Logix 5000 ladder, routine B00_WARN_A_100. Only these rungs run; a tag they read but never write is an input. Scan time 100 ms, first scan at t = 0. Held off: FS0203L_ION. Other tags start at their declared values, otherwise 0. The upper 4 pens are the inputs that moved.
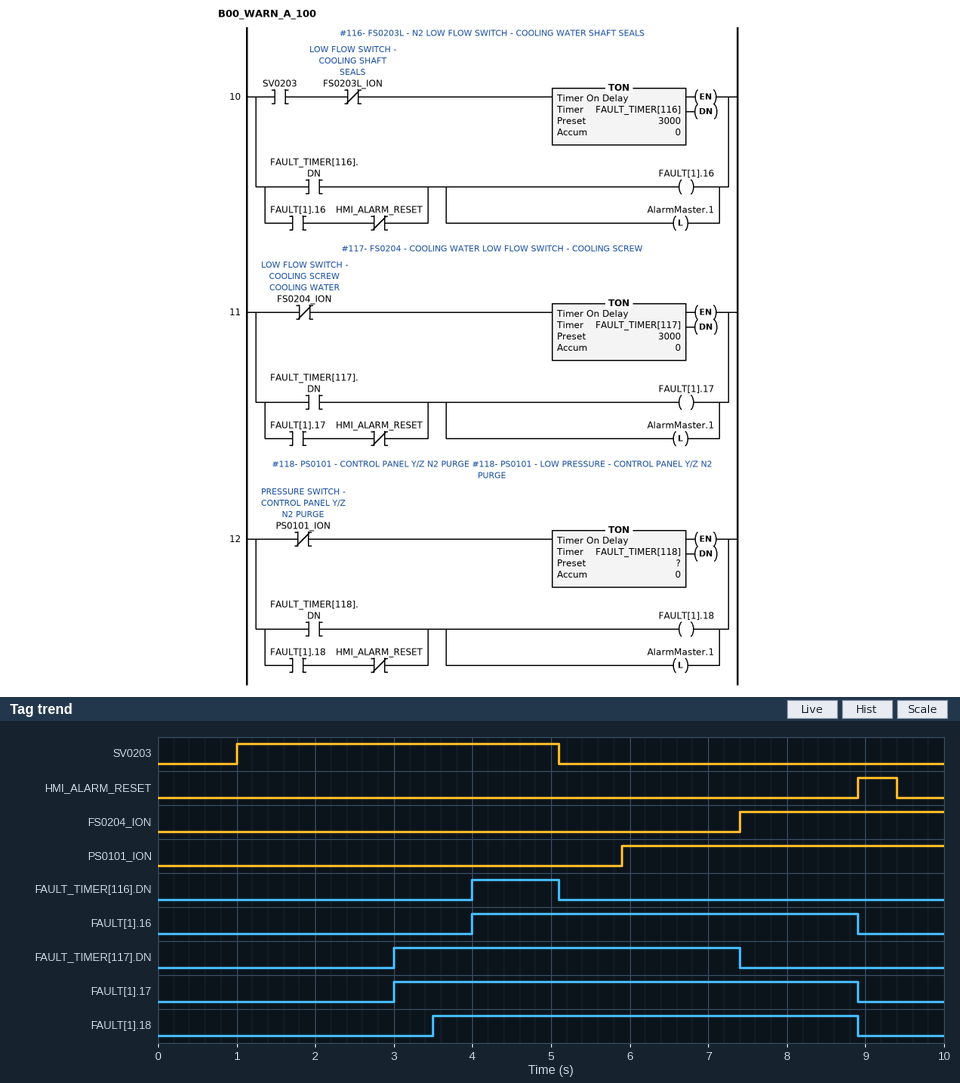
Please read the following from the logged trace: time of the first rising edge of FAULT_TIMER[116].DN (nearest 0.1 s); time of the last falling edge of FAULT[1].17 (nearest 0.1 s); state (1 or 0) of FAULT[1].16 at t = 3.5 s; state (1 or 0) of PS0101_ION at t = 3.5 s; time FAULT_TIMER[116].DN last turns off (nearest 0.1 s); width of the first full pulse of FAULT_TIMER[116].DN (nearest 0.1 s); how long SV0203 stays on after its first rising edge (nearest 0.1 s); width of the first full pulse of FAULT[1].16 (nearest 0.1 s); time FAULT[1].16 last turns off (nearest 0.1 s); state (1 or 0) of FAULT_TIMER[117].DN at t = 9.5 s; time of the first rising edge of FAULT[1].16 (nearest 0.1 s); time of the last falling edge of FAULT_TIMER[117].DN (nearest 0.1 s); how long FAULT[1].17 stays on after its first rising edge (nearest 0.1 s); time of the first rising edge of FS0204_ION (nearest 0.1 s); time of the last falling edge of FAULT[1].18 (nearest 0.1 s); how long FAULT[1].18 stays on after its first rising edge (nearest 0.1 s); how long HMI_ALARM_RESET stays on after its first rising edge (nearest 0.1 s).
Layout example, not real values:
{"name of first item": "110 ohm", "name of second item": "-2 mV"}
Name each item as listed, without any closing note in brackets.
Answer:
{"time of the first rising edge of FAULT_TIMER[116].DN": "4.0 s", "time of the last falling edge of FAULT[1].17": "8.9 s", "state (1 or 0) of FAULT[1].16 at t = 3.5 s": "0", "state (1 or 0) of PS0101_ION at t = 3.5 s": "0", "time FAULT_TIMER[116].DN last turns off": "5.1 s", "width of the first full pulse of FAULT_TIMER[116].DN": "1.1 s", "how long SV0203 stays on after its first rising edge": "4.1 s", "width of the first full pulse of FAULT[1].16": "4.9 s", "time FAULT[1].16 last turns off": "8.9 s", "state (1 or 0) of FAULT_TIMER[117].DN at t = 9.5 s": "0", "time of the first rising edge of FAULT[1].16": "4.0 s", "time of the last falling edge of FAULT_TIMER[117].DN": "7.4 s", "how long FAULT[1].17 stays on after its first rising edge": "5.9 s", "time of the first rising edge of FS0204_ION": "7.4 s", "time of the last falling edge of FAULT[1].18": "8.9 s", "how long FAULT[1].18 stays on after its first rising edge": "5.4 s", "how long HMI_ALARM_RESET stays on after its first rising edge": "0.5 s"}
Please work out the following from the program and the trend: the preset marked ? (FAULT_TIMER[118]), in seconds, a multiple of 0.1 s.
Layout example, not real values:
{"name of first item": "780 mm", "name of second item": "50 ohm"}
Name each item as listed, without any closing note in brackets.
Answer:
{"the preset marked ? (FAULT_TIMER[118]), in seconds, a multiple of 0.1 s": "3.5 s"}
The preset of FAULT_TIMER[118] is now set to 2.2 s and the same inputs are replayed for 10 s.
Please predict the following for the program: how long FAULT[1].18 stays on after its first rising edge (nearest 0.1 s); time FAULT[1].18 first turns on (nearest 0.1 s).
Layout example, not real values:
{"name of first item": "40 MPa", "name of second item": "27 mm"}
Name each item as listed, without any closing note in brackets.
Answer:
{"how long FAULT[1].18 stays on after its first rising edge": "6.7 s", "time FAULT[1].18 first turns on": "2.2 s"}
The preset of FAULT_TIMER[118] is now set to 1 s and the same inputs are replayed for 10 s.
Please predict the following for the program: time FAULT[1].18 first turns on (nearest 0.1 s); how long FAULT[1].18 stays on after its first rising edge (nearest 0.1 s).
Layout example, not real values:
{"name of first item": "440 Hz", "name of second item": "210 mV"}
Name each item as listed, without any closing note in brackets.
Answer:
{"time FAULT[1].18 first turns on": "1.0 s", "how long FAULT[1].18 stays on after its first rising edge": "7.9 s"}
